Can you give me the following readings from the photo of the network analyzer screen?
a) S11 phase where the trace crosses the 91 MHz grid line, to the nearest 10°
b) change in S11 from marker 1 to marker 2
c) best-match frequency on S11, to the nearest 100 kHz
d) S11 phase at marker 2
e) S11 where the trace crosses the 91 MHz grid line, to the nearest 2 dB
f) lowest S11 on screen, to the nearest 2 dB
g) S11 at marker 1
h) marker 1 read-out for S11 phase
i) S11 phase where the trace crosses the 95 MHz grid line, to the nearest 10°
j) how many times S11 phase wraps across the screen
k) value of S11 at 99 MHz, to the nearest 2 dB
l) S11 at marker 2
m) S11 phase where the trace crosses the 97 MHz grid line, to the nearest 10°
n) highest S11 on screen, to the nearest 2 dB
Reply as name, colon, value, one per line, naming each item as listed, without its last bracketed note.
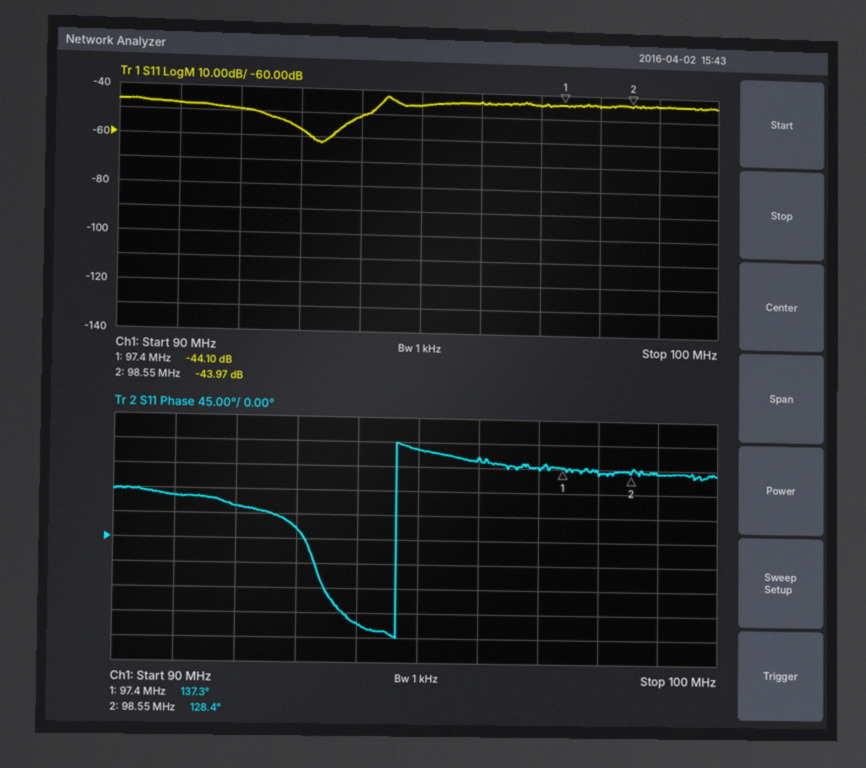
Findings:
S11 phase where the trace crosses the 91 MHz grid line, to the nearest 10°: 80°
change in S11 from marker 1 to marker 2: 0.13 dB
best-match frequency on S11, to the nearest 100 kHz: 93.3 MHz
S11 phase at marker 2: 128.4°
S11 where the trace crosses the 91 MHz grid line, to the nearest 2 dB: -48 dB
lowest S11 on screen, to the nearest 2 dB: -62 dB
S11 at marker 1: -44.10 dB
marker 1 read-out for S11 phase: 137.3°
S11 phase where the trace crosses the 95 MHz grid line, to the nearest 10°: 170°
how many times S11 phase wraps across the screen: 1
value of S11 at 99 MHz, to the nearest 2 dB: -44 dB
S11 at marker 2: -43.97 dB
S11 phase where the trace crosses the 97 MHz grid line, to the nearest 10°: 140°
highest S11 on screen, to the nearest 2 dB: -42 dB
